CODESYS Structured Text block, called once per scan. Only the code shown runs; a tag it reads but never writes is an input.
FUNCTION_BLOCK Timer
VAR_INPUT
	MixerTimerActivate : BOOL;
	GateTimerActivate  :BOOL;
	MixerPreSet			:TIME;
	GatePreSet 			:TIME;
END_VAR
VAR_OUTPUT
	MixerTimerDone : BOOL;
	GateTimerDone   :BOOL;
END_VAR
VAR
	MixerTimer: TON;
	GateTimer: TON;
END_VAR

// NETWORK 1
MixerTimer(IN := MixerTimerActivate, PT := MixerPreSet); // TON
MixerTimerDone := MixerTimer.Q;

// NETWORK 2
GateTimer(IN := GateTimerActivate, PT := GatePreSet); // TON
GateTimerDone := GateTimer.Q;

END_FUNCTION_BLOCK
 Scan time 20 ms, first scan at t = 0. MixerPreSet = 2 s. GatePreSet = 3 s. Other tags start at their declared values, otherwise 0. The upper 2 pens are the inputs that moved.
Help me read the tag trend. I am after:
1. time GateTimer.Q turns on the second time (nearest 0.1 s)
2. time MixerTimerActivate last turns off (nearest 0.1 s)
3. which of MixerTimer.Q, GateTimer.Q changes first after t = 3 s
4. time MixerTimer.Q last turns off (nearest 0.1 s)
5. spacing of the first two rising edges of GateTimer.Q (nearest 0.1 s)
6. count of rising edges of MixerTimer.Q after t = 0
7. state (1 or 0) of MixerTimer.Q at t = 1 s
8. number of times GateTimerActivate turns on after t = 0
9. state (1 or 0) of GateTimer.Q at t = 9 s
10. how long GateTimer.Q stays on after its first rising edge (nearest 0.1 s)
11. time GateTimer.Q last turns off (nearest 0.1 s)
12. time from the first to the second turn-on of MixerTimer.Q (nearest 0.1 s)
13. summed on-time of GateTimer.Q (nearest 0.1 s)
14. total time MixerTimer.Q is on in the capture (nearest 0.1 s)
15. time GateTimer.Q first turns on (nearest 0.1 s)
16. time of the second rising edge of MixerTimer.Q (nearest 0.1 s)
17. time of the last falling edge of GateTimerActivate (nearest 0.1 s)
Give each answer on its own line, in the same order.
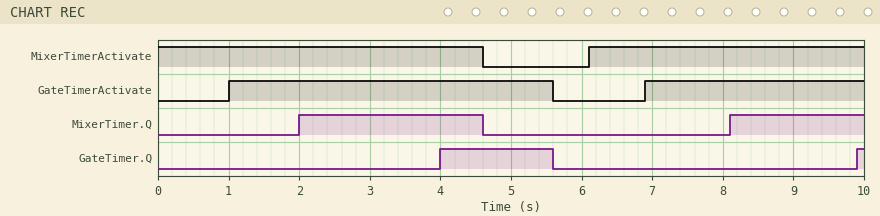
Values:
9.9 s
4.6 s
GateTimer.Q
4.6 s
5.9 s
2
0
2
0
1.6 s
5.6 s
6.1 s
1.7 s
4.5 s
4.0 s
8.1 s
5.6 s
